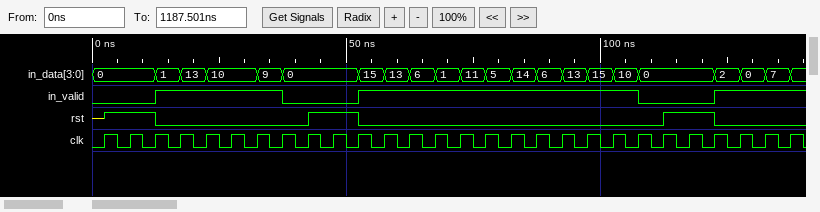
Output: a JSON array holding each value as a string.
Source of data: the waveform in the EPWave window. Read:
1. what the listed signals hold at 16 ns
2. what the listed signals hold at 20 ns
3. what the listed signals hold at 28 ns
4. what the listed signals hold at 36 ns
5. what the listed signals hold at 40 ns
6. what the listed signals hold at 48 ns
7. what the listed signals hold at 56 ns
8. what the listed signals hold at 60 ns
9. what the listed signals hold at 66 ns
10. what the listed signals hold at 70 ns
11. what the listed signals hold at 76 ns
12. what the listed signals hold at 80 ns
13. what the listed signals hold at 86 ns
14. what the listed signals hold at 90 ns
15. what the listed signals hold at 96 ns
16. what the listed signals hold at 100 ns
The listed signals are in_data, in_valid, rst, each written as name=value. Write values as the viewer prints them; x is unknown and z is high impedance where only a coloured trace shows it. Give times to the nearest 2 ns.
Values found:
["in_data=1, in_valid=1, rst=0", "in_data=13, in_valid=1, rst=0", "in_data=10, in_valid=1, rst=0", "in_data=9, in_valid=1, rst=0", "in_data=0, in_valid=0, rst=0", "in_data=0, in_valid=0, rst=1", "in_data=15, in_valid=1, rst=0", "in_data=13, in_valid=1, rst=0", "in_data=6, in_valid=1, rst=0", "in_data=1, in_valid=1, rst=0", "in_data=11, in_valid=1, rst=0", "in_data=5, in_valid=1, rst=0", "in_data=14, in_valid=1, rst=0", "in_data=6, in_valid=1, rst=0", "in_data=13, in_valid=1, rst=0", "in_data=15, in_valid=1, rst=0"]
